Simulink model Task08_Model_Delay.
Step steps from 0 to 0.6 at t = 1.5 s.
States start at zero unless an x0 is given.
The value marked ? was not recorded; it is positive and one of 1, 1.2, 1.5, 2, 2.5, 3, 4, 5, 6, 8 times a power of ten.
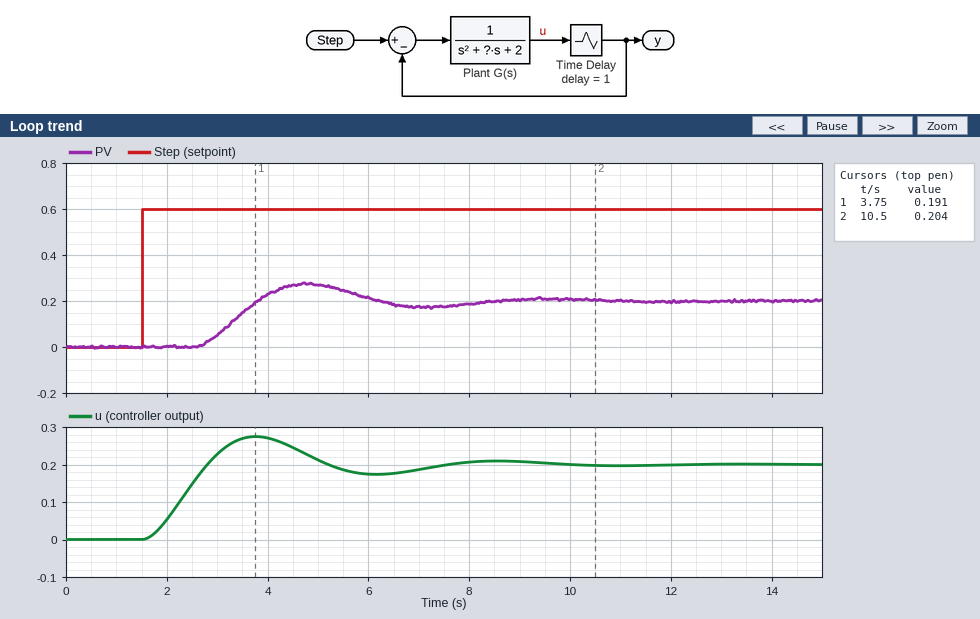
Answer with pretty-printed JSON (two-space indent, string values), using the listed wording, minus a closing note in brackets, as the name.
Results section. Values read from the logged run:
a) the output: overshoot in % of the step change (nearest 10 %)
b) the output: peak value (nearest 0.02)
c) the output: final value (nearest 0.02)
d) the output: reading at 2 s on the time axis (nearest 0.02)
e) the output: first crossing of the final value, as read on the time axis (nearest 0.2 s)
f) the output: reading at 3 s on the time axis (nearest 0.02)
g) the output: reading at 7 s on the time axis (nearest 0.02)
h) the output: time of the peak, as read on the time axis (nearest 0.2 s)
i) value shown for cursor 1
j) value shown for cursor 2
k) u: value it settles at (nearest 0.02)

{
  "the output: overshoot in % of the step change": "40 %",
  "the output: peak value": "0.28",
  "the output: final value": "0.20",
  "the output: reading at 2 s on the time axis": "0.00",
  "the output: first crossing of the final value, as read on the time axis": "3.8 s",
  "the output: reading at 3 s on the time axis": "0.06",
  "the output: reading at 7 s on the time axis": "0.18",
  "the output: time of the peak, as read on the time axis": "4.8 s",
  "value shown for cursor 1": "0.191",
  "value shown for cursor 2": "0.204",
  "u: value it settles at": "0.20"
}
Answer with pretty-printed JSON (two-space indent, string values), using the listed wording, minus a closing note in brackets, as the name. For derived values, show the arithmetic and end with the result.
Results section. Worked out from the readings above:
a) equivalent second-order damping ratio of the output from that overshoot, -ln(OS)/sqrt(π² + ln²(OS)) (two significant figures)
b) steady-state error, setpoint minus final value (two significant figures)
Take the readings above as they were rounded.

{
  "equivalent second-order damping ratio of the output from that overshoot, -ln(OS)/sqrt(π² + ln²(OS))": "ln(0.4) = -0.916; 0.916 / sqrt(9.870 + 0.840) = 0.28",
  "steady-state error, setpoint minus final value": "0.6 - 0.2 = 0.40"
}
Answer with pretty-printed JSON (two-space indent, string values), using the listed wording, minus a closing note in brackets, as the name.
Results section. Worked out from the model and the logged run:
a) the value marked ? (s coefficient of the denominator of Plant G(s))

{
  "the value marked ? (s coefficient of the denominator of Plant G(s))": "2"
}
